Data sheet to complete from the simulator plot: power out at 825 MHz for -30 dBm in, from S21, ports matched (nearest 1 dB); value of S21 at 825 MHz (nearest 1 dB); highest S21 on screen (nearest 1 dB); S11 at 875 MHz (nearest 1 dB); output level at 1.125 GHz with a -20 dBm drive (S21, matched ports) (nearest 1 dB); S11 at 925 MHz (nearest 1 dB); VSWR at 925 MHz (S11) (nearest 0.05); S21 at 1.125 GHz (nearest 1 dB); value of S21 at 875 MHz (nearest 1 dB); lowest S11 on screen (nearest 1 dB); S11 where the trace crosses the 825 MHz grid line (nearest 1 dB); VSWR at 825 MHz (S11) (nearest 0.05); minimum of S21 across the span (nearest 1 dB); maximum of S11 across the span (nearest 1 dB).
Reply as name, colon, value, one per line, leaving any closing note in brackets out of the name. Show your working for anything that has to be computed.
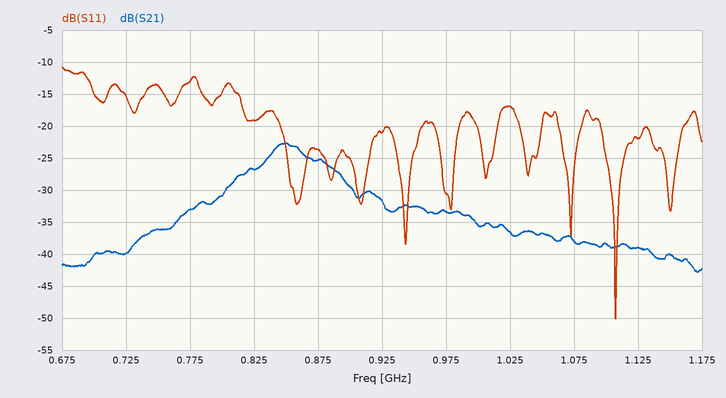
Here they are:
power out at 825 MHz for -30 dBm in, from S21, ports matched: -30 dBm + (-27 dB) = -57 dBm
value of S21 at 825 MHz: -27 dB
highest S21 on screen: -23 dB
S11 at 875 MHz: -24 dB
output level at 1.125 GHz with a -20 dBm drive (S21, matched ports): -20 dBm + (-39 dB) = -59 dBm
S11 at 925 MHz: -21 dB
VSWR at 925 MHz (S11): |Γ| = 10^(-21/20) = 0.0891; VSWR = (1 + 0.0891)/(1 − 0.0891) ≈ 1.20
S21 at 1.125 GHz: -39 dB
value of S21 at 875 MHz: -25 dB
lowest S11 on screen: -50 dB
S11 where the trace crosses the 825 MHz grid line: -19 dB
VSWR at 825 MHz (S11): |Γ| = 10^(-19/20) = 0.1122; VSWR = (1 + 0.1122)/(1 − 0.1122) ≈ 1.25
minimum of S21 across the span: -43 dB
maximum of S11 across the span: -11 dB
